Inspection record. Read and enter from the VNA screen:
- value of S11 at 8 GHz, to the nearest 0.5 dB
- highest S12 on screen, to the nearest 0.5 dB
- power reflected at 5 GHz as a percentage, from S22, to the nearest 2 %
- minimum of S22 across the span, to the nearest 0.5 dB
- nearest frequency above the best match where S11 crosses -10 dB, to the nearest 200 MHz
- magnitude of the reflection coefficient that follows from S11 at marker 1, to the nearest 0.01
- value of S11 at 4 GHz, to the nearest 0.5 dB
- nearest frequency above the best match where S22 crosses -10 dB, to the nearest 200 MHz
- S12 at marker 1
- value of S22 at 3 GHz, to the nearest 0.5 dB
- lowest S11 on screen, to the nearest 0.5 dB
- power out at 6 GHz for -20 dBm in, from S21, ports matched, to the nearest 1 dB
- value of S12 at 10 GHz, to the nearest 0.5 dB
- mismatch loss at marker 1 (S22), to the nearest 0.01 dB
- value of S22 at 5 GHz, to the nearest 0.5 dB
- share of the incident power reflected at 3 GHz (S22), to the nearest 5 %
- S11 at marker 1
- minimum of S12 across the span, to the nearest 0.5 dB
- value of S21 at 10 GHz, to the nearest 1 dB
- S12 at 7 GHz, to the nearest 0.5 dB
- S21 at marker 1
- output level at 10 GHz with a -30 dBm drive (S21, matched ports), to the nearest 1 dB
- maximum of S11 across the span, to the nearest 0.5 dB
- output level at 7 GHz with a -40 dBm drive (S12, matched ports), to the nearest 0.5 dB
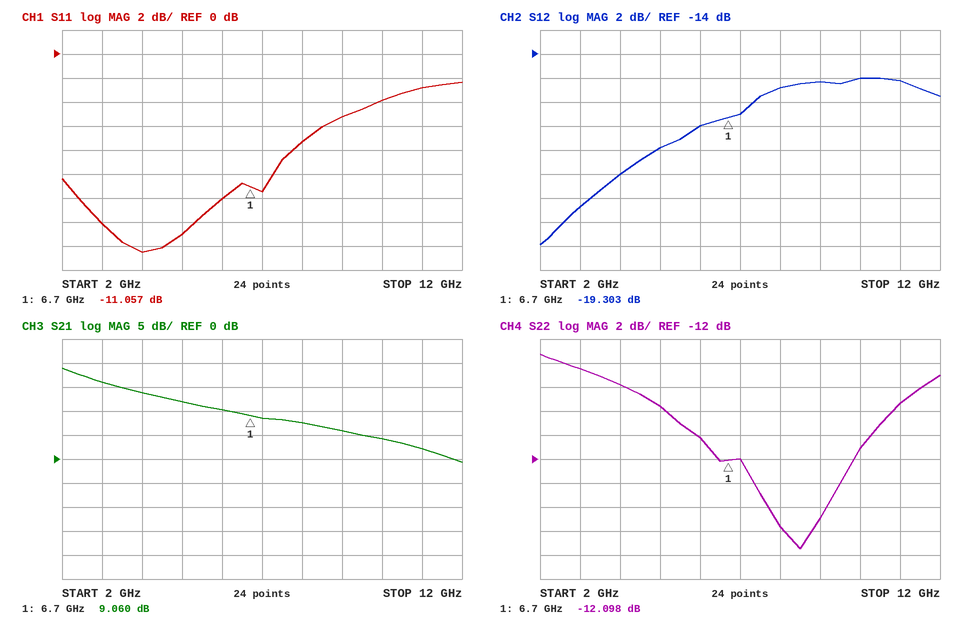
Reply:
-7.5 dB
-16.0 dB
18 %
-19.5 dB
7.2 GHz
0.28
-16.5 dB
10.2 GHz
-19.303 dB
-4.5 dB
-16.5 dB
-10 dBm
-16.0 dB
0.28 dB
-7.5 dB
35 %
-11.057 dB
-30.0 dB
4 dB
-19.0 dB
9.060 dB
-26 dBm
-2.5 dB
-59.0 dBm
